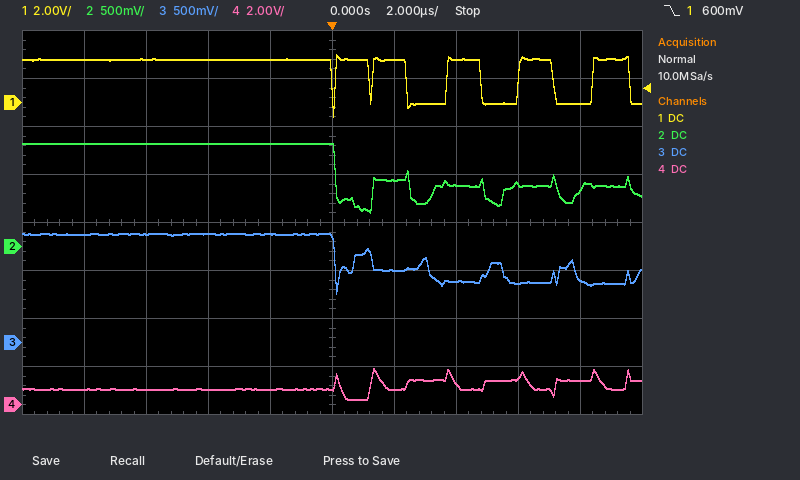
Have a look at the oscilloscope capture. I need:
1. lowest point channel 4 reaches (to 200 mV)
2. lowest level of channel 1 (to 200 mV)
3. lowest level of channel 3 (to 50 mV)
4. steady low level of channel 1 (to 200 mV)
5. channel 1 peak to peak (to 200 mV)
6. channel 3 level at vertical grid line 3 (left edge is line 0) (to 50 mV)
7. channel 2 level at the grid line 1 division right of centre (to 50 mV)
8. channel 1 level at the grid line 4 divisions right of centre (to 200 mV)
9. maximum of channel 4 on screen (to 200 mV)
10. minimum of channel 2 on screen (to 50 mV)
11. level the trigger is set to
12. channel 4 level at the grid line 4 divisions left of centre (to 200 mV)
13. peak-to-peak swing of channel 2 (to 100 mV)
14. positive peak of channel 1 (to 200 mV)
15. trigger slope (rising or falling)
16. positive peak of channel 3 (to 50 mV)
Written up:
200 mV
-600 mV
500 mV
0.0 V
2.6 V
1.15 V
700 mV
0.0 V
1.6 V
350 mV
600 mV
600 mV
700 mV
2.0 V
falling
1.15 V
